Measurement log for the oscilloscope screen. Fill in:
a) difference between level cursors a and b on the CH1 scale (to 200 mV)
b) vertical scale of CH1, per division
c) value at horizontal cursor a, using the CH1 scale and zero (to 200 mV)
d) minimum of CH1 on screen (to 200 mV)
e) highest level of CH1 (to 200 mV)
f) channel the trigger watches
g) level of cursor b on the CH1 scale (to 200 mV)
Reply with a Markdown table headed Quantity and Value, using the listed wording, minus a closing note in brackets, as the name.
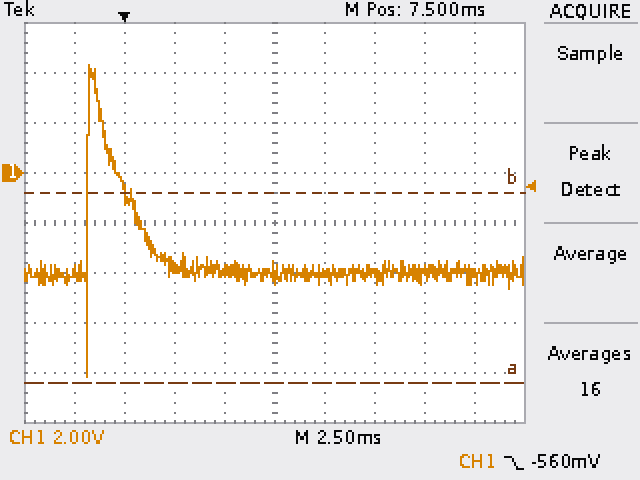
| Quantity | Value |
|---|---|
| difference between level cursors a and b on the CH1 scale | 7.6 V |
| vertical scale of CH1, per division | 2 V |
| value at horizontal cursor a, using the CH1 scale and zero | -8.4 V |
| minimum of CH1 on screen | -8.2 V |
| highest level of CH1 | 4.4 V |
| channel the trigger watches | CH1 |
| level of cursor b on the CH1 scale | -800 mV |
